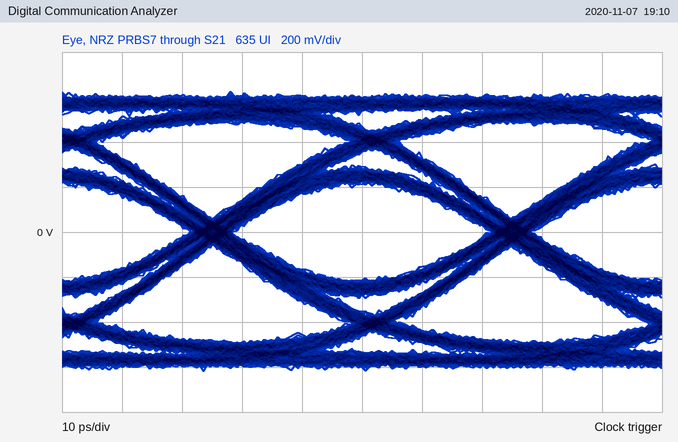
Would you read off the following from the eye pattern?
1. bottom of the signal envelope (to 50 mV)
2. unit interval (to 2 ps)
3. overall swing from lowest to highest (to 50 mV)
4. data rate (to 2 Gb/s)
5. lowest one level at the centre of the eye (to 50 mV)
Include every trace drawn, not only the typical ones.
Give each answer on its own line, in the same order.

-600 mV
50 ps
1.25 V
20 Gb/s
200 mV
